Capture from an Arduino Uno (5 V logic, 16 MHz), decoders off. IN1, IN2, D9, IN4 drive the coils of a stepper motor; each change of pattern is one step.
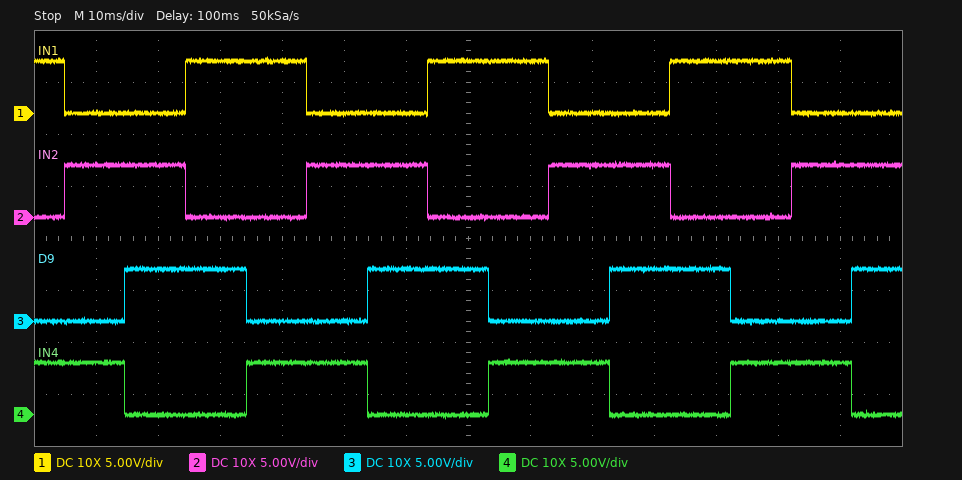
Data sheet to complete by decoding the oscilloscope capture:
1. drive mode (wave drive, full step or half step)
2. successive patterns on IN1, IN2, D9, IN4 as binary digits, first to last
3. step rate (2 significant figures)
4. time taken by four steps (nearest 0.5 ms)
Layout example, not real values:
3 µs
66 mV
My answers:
full step
1001 0101 0110 1010 1001 0101 0110 1010 1001 0101 0110 1010 1001 0101 0110
100 steps/s
39.0 ms
